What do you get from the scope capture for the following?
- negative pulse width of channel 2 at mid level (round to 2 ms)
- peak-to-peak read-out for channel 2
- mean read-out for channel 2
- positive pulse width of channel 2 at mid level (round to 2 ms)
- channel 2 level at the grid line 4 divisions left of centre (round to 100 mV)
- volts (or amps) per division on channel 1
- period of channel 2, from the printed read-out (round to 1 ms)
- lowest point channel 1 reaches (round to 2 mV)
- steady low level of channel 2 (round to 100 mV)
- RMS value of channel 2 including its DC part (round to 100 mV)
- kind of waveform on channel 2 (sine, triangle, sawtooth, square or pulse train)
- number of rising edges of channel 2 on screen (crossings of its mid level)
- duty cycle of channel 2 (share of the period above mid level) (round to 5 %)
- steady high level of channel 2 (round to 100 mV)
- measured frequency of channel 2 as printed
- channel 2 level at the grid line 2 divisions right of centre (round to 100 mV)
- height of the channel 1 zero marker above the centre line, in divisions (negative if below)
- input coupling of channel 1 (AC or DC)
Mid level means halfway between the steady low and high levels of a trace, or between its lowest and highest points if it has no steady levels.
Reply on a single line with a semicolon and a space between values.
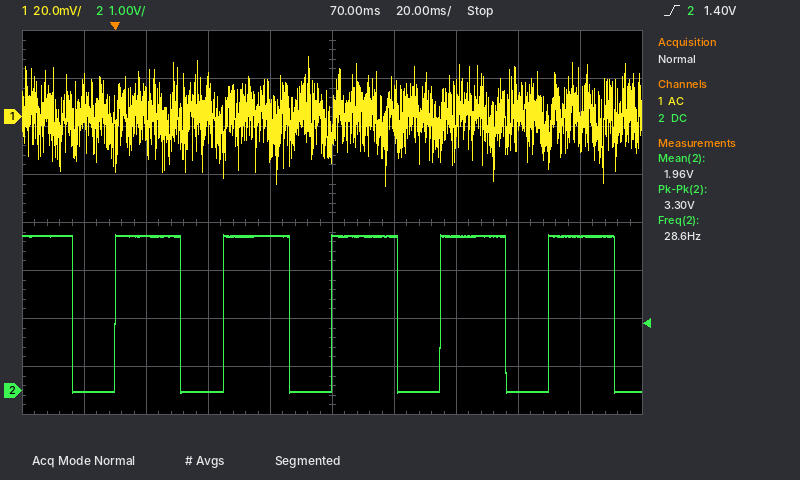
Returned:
14 ms; 3.30 V; 1.96 V; 22 ms; 0.0 V; 20 mV; 35 ms; -28 mV; 0.0 V; 2.5 V; pulse train; 5; 60 %; 3.2 V; 28.6 Hz; 3.2 V; +2.2 div; AC
